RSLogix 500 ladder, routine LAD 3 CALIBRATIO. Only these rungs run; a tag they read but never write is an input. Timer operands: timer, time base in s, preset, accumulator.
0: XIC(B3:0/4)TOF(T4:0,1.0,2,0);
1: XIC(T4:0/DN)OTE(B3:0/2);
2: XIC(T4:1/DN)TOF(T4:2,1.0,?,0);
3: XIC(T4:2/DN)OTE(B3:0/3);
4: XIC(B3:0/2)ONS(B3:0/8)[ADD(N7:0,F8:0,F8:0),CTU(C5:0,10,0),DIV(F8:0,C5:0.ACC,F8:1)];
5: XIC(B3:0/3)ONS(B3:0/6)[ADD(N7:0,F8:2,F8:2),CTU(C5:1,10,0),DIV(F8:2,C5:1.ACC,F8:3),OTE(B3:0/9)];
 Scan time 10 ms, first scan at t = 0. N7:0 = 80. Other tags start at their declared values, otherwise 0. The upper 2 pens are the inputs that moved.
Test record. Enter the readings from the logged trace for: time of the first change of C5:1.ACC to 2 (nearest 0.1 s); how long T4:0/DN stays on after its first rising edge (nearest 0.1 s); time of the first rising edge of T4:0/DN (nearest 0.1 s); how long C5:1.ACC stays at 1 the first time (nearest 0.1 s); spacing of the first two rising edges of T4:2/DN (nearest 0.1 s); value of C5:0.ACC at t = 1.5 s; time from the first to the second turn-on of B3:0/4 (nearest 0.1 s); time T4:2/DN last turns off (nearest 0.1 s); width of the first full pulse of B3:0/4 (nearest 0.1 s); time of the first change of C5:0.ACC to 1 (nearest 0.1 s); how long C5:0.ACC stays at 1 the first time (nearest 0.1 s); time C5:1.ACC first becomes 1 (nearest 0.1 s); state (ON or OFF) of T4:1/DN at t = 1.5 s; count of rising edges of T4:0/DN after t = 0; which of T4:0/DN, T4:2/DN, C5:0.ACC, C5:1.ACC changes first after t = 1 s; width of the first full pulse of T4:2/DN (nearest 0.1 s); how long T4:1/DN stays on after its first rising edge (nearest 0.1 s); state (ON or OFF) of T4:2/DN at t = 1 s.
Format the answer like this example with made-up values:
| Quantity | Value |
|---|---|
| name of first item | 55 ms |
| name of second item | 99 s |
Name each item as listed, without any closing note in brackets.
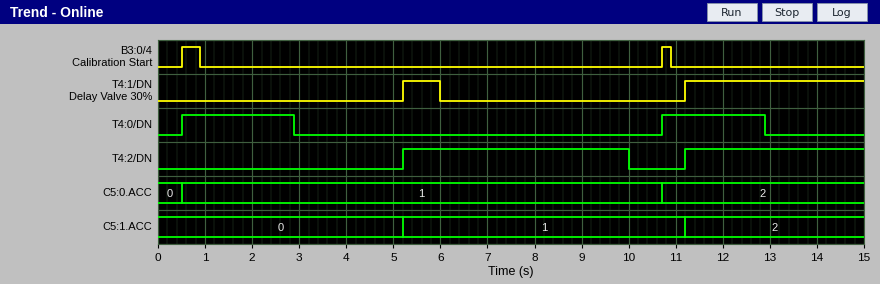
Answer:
| Quantity | Value |
|---|---|
| time of the first change of C5:1.ACC to 2 | 11.2 s |
| how long T4:0/DN stays on after its first rising edge | 2.4 s |
| time of the first rising edge of T4:0/DN | 0.5 s |
| how long C5:1.ACC stays at 1 the first time | 6.0 s |
| spacing of the first two rising edges of T4:2/DN | 6.0 s |
| value of C5:0.ACC at t = 1.5 s | 1 |
| time from the first to the second turn-on of B3:0/4 | 10.2 s |
| time T4:2/DN last turns off | 10.0 s |
| width of the first full pulse of B3:0/4 | 0.4 s |
| time of the first change of C5:0.ACC to 1 | 0.5 s |
| how long C5:0.ACC stays at 1 the first time | 10.2 s |
| time C5:1.ACC first becomes 1 | 5.2 s |
| state (ON or OFF) of T4:1/DN at t = 1.5 s | OFF |
| count of rising edges of T4:0/DN after t = 0 | 2 |
| which of T4:0/DN, T4:2/DN, C5:0.ACC, C5:1.ACC changes first after t = 1 s | T4:0/DN |
| width of the first full pulse of T4:2/DN | 4.8 s |
| how long T4:1/DN stays on after its first rising edge | 0.8 s |
| state (ON or OFF) of T4:2/DN at t = 1 s | OFF |
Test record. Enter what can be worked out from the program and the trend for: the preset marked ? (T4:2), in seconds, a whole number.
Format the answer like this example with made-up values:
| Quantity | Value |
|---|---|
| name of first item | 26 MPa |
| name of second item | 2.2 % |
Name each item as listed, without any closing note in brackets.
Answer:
| Quantity | Value |
|---|---|
| the preset marked ? (T4:2), in seconds, a whole number | 4 s |
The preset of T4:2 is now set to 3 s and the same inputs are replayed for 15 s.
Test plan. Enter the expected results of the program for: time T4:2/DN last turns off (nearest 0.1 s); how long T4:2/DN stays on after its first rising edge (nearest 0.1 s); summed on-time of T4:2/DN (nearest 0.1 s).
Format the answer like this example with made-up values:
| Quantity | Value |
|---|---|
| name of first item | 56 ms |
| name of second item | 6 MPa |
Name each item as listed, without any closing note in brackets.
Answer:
| Quantity | Value |
|---|---|
| time T4:2/DN last turns off | 9.0 s |
| how long T4:2/DN stays on after its first rising edge | 3.8 s |
| summed on-time of T4:2/DN | 7.6 s |
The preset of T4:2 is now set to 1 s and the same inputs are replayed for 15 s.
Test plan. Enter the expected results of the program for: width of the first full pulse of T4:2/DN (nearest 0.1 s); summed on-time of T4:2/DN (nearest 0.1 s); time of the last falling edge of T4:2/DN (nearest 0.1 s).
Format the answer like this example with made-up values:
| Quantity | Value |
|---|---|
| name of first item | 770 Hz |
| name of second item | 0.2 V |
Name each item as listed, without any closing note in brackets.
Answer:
| Quantity | Value |
|---|---|
| width of the first full pulse of T4:2/DN | 1.8 s |
| summed on-time of T4:2/DN | 5.6 s |
| time of the last falling edge of T4:2/DN | 7.0 s |
